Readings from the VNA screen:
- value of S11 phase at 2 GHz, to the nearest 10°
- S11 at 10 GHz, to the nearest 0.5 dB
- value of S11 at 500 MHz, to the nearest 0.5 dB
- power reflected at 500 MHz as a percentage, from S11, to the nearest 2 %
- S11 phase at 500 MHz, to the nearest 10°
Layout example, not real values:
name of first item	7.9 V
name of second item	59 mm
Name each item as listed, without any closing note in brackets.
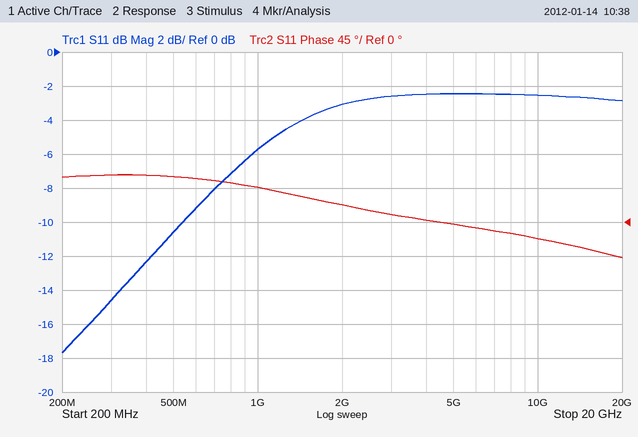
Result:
value of S11 phase at 2 GHz, to the nearest 10°	20°
S11 at 10 GHz, to the nearest 0.5 dB	-2.5 dB
value of S11 at 500 MHz, to the nearest 0.5 dB	-10.5 dB
power reflected at 500 MHz as a percentage, from S11, to the nearest 2 %	8 %
S11 phase at 500 MHz, to the nearest 10°	60°
